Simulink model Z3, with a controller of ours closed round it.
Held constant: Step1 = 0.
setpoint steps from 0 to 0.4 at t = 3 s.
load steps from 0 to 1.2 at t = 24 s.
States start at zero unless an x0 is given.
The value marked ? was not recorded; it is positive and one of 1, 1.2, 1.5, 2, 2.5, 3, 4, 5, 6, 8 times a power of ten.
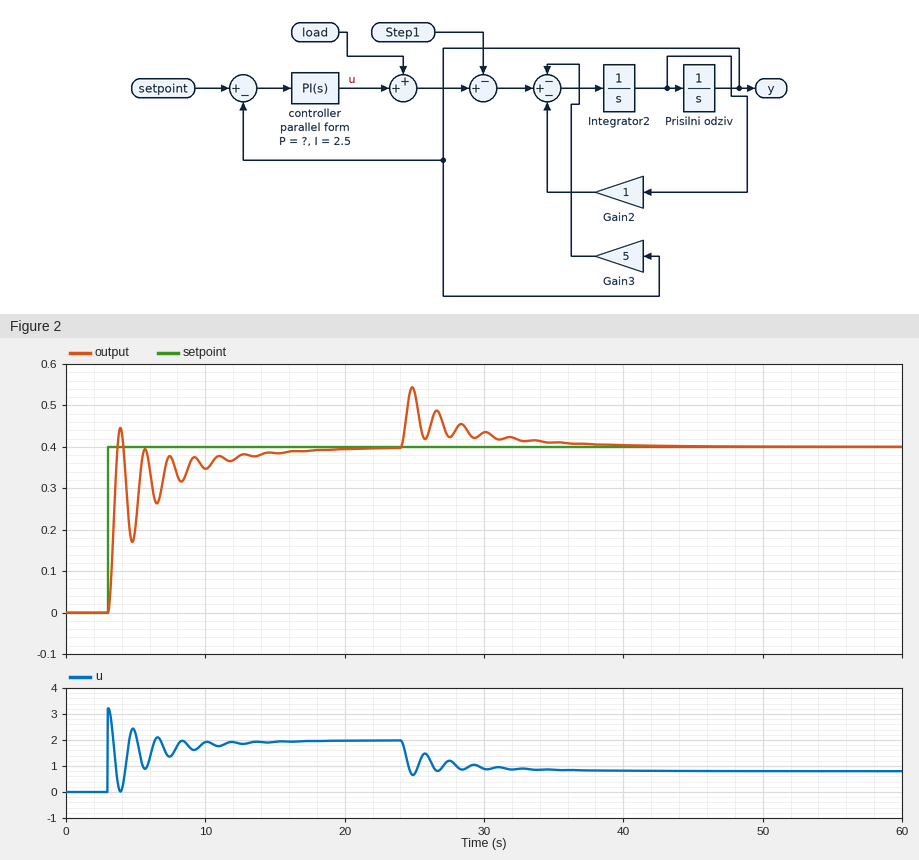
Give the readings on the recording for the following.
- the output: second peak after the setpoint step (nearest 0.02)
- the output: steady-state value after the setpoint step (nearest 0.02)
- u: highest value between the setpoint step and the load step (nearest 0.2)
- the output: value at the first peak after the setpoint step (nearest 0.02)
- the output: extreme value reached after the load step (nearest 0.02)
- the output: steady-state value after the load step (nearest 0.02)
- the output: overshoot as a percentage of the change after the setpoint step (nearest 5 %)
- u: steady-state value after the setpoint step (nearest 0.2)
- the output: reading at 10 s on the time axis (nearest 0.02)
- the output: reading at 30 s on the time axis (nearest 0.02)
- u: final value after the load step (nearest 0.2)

0.40
0.40
3.2
0.44
0.54
0.40
10 %
2.0
0.34
0.44
0.8
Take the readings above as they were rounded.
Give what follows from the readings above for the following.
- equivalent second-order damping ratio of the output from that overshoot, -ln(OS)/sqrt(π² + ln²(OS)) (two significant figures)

0.59
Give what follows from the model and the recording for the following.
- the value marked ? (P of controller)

8
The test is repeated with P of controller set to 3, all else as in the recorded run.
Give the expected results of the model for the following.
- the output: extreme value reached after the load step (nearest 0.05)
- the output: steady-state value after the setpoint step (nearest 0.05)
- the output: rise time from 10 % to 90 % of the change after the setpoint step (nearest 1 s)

0.60
0.40
3 s
